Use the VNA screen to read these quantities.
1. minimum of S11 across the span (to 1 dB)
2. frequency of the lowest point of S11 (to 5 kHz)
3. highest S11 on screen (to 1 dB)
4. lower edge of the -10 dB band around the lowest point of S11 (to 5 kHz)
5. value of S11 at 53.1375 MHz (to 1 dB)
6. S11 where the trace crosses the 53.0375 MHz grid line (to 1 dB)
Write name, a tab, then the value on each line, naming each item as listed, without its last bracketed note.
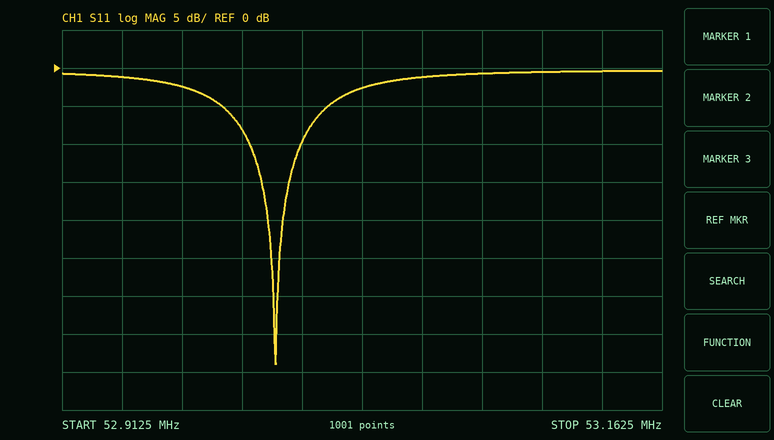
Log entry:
minimum of S11 across the span	-39 dB
frequency of the lowest point of S11	53.000 MHz
highest S11 on screen	0 dB
lower edge of the -10 dB band around the lowest point of S11	52.990 MHz
value of S11 at 53.1375 MHz	0 dB
S11 where the trace crosses the 53.0375 MHz grid line	-3 dB
